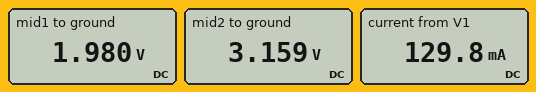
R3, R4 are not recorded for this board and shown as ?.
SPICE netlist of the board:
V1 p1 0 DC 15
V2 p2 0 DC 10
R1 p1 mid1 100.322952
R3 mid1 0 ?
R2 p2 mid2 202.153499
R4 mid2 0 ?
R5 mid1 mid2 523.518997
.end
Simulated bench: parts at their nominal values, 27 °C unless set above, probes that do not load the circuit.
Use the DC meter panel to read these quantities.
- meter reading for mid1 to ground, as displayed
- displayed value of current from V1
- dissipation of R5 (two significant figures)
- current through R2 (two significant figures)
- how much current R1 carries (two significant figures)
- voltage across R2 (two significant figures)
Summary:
1.980 V
129.8 mA
2.7 mW
34 mA
130 mA
6.8 V
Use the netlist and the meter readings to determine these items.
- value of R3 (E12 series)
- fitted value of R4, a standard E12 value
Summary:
15 Ω
100 Ω
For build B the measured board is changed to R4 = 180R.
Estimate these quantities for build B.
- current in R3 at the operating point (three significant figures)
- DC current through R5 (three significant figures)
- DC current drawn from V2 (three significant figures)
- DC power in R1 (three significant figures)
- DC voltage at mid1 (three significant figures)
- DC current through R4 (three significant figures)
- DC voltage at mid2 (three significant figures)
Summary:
134 mA
4.37 mA
28.2 mA
1.68 W
2.01 V
23.9 mA
4.29 V
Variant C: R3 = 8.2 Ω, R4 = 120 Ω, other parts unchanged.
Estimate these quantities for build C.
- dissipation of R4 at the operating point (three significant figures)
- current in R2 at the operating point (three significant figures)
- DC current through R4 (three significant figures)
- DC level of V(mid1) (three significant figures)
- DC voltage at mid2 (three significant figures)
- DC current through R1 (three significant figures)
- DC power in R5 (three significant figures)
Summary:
96.5 mW
32.6 mA
28.4 mA
1.17 V
3.40 V
138 mA
9.56 mW
